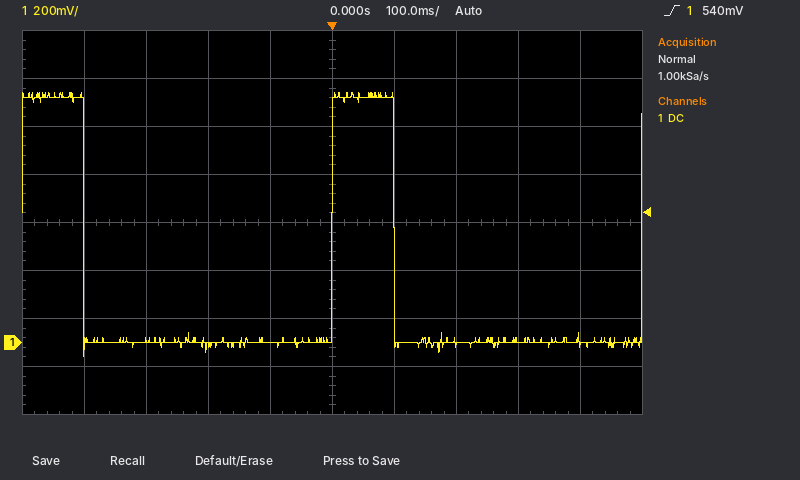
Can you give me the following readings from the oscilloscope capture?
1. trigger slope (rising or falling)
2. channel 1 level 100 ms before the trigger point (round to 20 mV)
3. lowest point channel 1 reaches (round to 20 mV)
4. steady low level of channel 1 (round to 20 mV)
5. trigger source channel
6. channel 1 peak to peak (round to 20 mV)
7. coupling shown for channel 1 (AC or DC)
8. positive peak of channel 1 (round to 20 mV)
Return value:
rising
0 mV
-60 mV
0 mV
channel 1
1.10 V
DC
1.04 V
